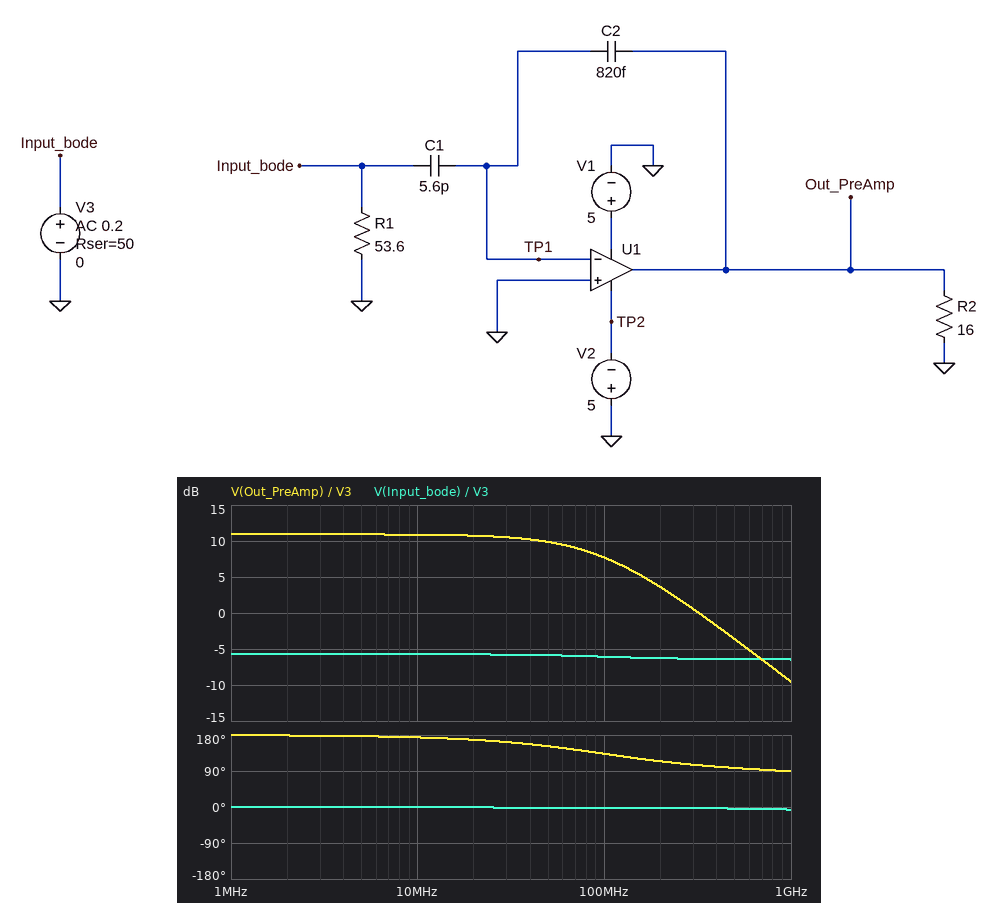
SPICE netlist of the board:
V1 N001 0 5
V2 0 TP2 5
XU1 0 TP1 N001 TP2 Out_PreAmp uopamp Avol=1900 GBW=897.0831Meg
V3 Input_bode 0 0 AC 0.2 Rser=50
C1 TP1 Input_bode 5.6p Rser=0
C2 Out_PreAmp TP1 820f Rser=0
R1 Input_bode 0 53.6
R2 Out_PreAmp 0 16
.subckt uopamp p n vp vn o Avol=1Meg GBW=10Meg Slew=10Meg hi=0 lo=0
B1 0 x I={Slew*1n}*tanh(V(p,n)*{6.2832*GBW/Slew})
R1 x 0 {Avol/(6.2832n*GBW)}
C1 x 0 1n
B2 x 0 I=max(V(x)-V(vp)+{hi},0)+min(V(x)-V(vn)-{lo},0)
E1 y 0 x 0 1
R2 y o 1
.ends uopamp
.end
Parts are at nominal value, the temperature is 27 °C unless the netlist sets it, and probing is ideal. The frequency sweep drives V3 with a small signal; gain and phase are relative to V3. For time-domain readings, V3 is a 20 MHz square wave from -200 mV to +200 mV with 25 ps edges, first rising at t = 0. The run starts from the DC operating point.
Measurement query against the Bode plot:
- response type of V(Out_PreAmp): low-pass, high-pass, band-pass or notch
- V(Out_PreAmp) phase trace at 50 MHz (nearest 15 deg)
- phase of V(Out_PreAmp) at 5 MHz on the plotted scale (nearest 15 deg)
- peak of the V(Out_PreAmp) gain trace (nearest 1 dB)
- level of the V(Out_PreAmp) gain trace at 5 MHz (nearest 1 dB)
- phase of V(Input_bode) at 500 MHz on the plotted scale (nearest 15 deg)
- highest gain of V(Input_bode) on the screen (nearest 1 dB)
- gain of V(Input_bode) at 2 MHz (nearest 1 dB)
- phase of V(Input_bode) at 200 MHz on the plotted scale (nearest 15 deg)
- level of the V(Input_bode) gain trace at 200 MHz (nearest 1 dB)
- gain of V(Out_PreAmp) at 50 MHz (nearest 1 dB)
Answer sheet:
low-pass
150 deg
180 deg
11 dB
11 dB
0 deg
-6 dB
-6 dB
0 deg
-6 dB
10 dB
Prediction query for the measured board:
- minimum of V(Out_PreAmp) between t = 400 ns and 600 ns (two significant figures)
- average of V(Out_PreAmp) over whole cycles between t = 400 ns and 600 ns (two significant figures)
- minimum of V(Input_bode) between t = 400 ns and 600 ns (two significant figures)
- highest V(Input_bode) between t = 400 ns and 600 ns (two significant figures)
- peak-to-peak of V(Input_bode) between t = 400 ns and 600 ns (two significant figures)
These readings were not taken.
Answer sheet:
-230 mV
-110 mV
-100 mV
100 mV
210 mV
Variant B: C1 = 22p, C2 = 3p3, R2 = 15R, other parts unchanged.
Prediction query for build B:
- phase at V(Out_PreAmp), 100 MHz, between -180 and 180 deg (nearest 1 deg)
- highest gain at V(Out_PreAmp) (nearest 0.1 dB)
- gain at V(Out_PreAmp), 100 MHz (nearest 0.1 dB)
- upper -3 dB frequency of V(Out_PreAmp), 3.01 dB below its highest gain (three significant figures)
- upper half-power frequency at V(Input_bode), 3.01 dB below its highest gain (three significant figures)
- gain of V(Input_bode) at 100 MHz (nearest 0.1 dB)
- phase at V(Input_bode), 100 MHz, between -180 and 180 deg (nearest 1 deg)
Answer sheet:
127 deg
10.7 dB
6.7 dB
81.4 MHz
869 MHz
-7.1 dB
-11 deg
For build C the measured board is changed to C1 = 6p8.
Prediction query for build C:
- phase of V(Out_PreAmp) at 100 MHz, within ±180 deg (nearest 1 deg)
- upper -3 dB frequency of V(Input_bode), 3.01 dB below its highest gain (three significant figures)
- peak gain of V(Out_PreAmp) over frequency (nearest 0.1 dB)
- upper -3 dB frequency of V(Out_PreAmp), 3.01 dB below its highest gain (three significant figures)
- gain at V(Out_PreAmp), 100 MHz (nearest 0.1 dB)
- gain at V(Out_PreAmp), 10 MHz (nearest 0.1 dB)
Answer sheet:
129 deg
7.31 GHz
12.6 dB
83.8 MHz
8.8 dB
12.5 dB
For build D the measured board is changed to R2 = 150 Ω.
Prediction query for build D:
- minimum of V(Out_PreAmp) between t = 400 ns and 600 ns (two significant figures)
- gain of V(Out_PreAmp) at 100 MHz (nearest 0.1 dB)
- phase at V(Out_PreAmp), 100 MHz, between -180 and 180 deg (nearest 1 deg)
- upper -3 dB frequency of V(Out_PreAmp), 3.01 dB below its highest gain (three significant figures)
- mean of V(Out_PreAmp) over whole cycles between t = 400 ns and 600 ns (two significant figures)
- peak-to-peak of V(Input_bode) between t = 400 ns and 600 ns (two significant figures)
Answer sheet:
-250 mV
8.1 dB
136 deg
105 MHz
-120 mV
210 mV
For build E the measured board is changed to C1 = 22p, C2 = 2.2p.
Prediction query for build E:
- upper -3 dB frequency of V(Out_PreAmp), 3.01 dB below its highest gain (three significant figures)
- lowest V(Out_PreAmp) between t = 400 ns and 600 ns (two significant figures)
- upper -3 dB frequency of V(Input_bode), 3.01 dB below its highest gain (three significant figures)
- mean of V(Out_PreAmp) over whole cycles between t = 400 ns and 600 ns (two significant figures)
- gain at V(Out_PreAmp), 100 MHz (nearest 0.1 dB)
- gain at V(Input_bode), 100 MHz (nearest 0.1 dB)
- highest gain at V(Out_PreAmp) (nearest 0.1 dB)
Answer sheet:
61.6 MHz
-240 mV
1.94 GHz
-120 mV
8.6 dB
-7.1 dB
14.2 dB
